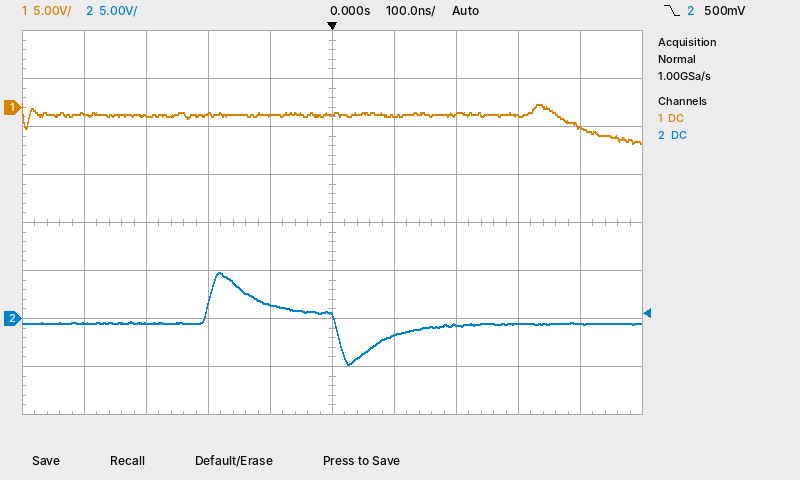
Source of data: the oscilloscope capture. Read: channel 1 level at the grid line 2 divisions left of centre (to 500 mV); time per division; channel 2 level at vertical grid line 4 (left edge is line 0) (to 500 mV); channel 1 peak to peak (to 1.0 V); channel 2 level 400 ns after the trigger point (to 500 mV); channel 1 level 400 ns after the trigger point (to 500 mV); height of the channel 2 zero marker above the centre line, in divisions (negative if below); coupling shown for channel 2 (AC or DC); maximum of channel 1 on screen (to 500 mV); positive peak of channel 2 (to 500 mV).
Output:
-500 mV
100 ns
1.5 V
4.0 V
-500 mV
-2.0 V
-2.0 div
DC
500 mV
5.0 V
